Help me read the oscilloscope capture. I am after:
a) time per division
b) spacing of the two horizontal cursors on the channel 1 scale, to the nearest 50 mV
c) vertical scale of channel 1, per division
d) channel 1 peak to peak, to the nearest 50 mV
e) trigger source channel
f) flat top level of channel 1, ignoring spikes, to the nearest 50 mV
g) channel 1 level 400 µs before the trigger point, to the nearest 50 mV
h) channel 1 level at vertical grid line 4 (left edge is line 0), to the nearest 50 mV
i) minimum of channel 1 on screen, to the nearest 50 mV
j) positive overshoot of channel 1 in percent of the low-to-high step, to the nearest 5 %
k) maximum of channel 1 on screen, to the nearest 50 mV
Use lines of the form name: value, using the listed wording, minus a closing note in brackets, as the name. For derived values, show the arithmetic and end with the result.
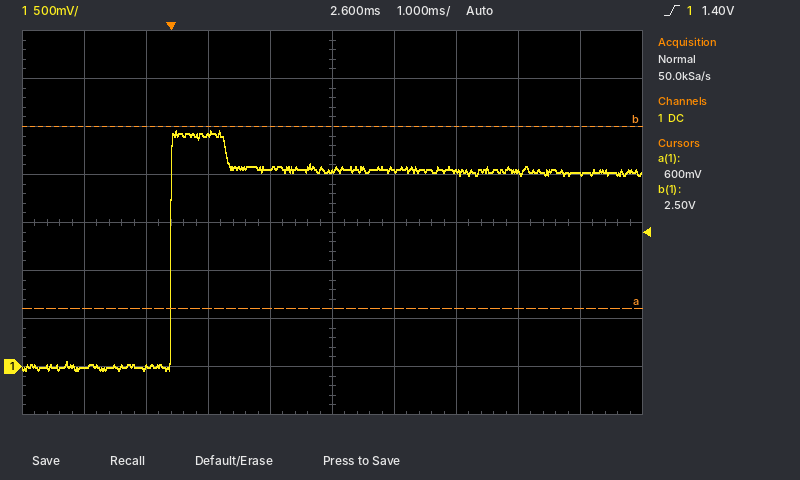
time per division: 1 ms
spacing of the two horizontal cursors on the channel 1 scale, to the nearest 50 mV: 1.90 V
vertical scale of channel 1, per division: 500 mV
channel 1 peak to peak, to the nearest 50 mV: 2.45 V − (-50 mV) = 2.50 V
trigger source channel: channel 1
flat top level of channel 1, ignoring spikes, to the nearest 50 mV: 2.05 V
channel 1 level 400 µs before the trigger point, to the nearest 50 mV: 0 mV
channel 1 level at vertical grid line 4 (left edge is line 0), to the nearest 50 mV: 2.05 V
minimum of channel 1 on screen, to the nearest 50 mV: -50 mV
positive overshoot of channel 1 in percent of the low-to-high step, to the nearest 5 %: 20 %
maximum of channel 1 on screen, to the nearest 50 mV: 2.45 V
